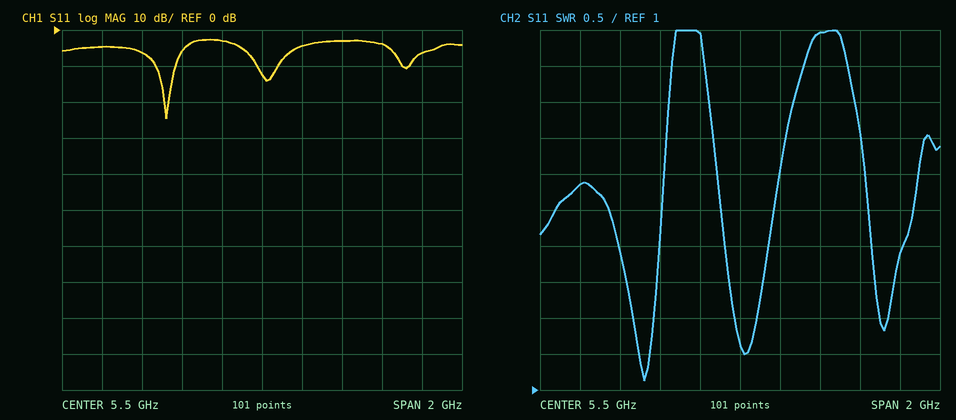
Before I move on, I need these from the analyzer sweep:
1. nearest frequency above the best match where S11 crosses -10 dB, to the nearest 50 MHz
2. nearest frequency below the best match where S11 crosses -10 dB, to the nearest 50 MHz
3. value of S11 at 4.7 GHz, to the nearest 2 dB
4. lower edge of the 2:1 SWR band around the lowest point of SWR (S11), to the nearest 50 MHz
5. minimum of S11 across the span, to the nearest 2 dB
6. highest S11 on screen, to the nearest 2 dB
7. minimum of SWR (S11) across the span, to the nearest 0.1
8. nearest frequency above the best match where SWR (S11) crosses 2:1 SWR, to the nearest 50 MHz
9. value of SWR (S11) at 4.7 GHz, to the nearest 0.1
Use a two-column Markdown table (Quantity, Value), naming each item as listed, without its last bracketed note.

| Quantity | Value |
|---|---|
| nearest frequency above the best match where S11 crosses -10 dB, to the nearest 50 MHz | 5.05 GHz |
| nearest frequency below the best match where S11 crosses -10 dB, to the nearest 50 MHz | 4.95 GHz |
| value of S11 at 4.7 GHz, to the nearest 2 dB | -4 dB |
| lower edge of the 2:1 SWR band around the lowest point of SWR (S11), to the nearest 50 MHz | 4.95 GHz |
| minimum of S11 across the span, to the nearest 2 dB | -24 dB |
| highest S11 on screen, to the nearest 2 dB | -2 dB |
| minimum of SWR (S11) across the span, to the nearest 0.1 | 1.1 |
| nearest frequency above the best match where SWR (S11) crosses 2:1 SWR, to the nearest 50 MHz | 5.05 GHz |
| value of SWR (S11) at 4.7 GHz, to the nearest 0.1 | 3.9 |
